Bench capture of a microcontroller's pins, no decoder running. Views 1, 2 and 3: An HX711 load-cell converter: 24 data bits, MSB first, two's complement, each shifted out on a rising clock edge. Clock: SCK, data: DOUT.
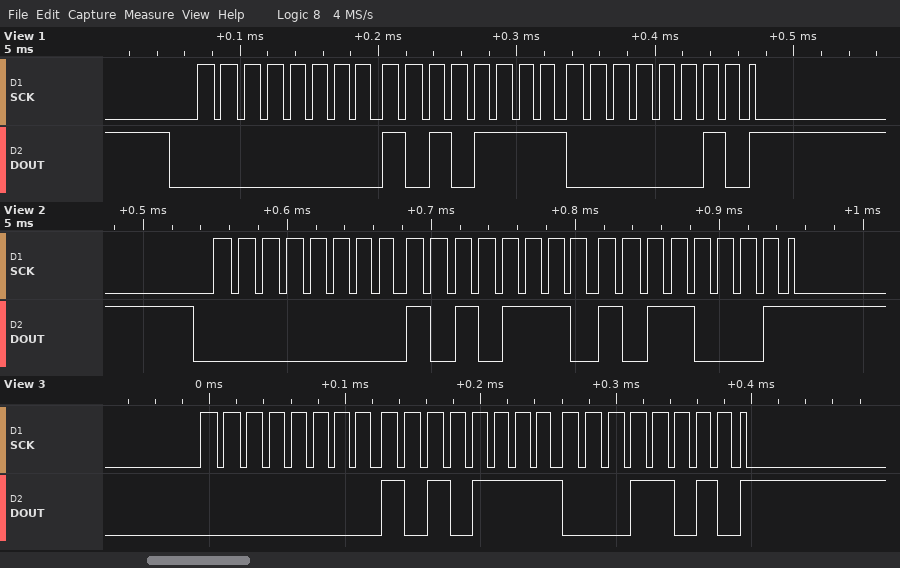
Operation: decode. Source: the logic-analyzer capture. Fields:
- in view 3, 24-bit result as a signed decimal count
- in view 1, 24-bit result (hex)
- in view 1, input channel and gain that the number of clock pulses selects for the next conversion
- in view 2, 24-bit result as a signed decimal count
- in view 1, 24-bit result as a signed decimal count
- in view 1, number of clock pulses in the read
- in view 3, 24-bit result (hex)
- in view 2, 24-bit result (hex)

44826
0x00AF02
channel A, gain 128
44721
44802
25
0x00AF1A
0x00AEB1
